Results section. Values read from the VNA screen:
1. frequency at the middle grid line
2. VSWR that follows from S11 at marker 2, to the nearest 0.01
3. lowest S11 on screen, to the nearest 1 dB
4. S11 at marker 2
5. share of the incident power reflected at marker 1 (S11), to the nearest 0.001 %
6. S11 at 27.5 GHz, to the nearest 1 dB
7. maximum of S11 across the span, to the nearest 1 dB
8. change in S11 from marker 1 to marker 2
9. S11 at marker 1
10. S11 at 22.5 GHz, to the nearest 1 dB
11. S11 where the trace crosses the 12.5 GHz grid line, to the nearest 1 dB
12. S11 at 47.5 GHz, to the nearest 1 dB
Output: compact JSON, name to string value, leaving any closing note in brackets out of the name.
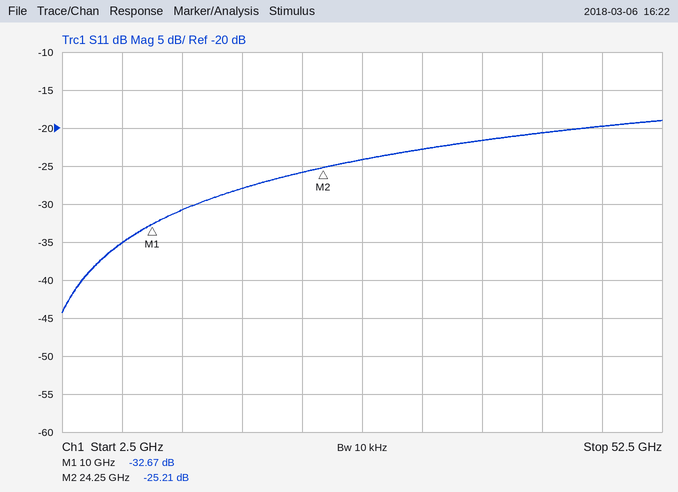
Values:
{"frequency at the middle grid line": "27.5 GHz", "VSWR that follows from S11 at marker 2, to the nearest 0.01": "1.12", "lowest S11 on screen, to the nearest 1 dB": "-44 dB", "S11 at marker 2": "-25.21 dB", "share of the incident power reflected at marker 1 (S11), to the nearest 0.001 %": "0.054 %", "S11 at 27.5 GHz, to the nearest 1 dB": "-24 dB", "maximum of S11 across the span, to the nearest 1 dB": "-19 dB", "change in S11 from marker 1 to marker 2": "7.46 dB", "S11 at marker 1": "-32.67 dB", "S11 at 22.5 GHz, to the nearest 1 dB": "-26 dB", "S11 where the trace crosses the 12.5 GHz grid line, to the nearest 1 dB": "-31 dB", "S11 at 47.5 GHz, to the nearest 1 dB": "-20 dB"}
